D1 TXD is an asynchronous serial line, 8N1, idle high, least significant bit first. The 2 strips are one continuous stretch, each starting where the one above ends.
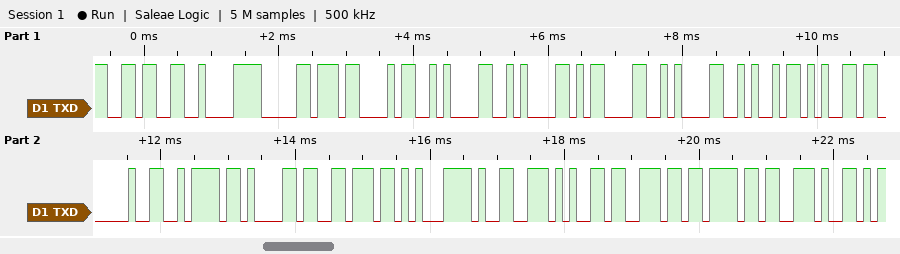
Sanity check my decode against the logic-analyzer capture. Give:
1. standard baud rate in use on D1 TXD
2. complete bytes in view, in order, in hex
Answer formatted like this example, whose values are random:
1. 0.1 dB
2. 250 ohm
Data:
1. 9600 baud
2. 0x36 0xC2 0xB0 0x43 0x0A 0x0A 0x0D 0x0A 0x4A 0x65 0x20 0x7A 0x61 0x76 0xC5 0x99 0x65 0x6E 0x6F 0x2E
